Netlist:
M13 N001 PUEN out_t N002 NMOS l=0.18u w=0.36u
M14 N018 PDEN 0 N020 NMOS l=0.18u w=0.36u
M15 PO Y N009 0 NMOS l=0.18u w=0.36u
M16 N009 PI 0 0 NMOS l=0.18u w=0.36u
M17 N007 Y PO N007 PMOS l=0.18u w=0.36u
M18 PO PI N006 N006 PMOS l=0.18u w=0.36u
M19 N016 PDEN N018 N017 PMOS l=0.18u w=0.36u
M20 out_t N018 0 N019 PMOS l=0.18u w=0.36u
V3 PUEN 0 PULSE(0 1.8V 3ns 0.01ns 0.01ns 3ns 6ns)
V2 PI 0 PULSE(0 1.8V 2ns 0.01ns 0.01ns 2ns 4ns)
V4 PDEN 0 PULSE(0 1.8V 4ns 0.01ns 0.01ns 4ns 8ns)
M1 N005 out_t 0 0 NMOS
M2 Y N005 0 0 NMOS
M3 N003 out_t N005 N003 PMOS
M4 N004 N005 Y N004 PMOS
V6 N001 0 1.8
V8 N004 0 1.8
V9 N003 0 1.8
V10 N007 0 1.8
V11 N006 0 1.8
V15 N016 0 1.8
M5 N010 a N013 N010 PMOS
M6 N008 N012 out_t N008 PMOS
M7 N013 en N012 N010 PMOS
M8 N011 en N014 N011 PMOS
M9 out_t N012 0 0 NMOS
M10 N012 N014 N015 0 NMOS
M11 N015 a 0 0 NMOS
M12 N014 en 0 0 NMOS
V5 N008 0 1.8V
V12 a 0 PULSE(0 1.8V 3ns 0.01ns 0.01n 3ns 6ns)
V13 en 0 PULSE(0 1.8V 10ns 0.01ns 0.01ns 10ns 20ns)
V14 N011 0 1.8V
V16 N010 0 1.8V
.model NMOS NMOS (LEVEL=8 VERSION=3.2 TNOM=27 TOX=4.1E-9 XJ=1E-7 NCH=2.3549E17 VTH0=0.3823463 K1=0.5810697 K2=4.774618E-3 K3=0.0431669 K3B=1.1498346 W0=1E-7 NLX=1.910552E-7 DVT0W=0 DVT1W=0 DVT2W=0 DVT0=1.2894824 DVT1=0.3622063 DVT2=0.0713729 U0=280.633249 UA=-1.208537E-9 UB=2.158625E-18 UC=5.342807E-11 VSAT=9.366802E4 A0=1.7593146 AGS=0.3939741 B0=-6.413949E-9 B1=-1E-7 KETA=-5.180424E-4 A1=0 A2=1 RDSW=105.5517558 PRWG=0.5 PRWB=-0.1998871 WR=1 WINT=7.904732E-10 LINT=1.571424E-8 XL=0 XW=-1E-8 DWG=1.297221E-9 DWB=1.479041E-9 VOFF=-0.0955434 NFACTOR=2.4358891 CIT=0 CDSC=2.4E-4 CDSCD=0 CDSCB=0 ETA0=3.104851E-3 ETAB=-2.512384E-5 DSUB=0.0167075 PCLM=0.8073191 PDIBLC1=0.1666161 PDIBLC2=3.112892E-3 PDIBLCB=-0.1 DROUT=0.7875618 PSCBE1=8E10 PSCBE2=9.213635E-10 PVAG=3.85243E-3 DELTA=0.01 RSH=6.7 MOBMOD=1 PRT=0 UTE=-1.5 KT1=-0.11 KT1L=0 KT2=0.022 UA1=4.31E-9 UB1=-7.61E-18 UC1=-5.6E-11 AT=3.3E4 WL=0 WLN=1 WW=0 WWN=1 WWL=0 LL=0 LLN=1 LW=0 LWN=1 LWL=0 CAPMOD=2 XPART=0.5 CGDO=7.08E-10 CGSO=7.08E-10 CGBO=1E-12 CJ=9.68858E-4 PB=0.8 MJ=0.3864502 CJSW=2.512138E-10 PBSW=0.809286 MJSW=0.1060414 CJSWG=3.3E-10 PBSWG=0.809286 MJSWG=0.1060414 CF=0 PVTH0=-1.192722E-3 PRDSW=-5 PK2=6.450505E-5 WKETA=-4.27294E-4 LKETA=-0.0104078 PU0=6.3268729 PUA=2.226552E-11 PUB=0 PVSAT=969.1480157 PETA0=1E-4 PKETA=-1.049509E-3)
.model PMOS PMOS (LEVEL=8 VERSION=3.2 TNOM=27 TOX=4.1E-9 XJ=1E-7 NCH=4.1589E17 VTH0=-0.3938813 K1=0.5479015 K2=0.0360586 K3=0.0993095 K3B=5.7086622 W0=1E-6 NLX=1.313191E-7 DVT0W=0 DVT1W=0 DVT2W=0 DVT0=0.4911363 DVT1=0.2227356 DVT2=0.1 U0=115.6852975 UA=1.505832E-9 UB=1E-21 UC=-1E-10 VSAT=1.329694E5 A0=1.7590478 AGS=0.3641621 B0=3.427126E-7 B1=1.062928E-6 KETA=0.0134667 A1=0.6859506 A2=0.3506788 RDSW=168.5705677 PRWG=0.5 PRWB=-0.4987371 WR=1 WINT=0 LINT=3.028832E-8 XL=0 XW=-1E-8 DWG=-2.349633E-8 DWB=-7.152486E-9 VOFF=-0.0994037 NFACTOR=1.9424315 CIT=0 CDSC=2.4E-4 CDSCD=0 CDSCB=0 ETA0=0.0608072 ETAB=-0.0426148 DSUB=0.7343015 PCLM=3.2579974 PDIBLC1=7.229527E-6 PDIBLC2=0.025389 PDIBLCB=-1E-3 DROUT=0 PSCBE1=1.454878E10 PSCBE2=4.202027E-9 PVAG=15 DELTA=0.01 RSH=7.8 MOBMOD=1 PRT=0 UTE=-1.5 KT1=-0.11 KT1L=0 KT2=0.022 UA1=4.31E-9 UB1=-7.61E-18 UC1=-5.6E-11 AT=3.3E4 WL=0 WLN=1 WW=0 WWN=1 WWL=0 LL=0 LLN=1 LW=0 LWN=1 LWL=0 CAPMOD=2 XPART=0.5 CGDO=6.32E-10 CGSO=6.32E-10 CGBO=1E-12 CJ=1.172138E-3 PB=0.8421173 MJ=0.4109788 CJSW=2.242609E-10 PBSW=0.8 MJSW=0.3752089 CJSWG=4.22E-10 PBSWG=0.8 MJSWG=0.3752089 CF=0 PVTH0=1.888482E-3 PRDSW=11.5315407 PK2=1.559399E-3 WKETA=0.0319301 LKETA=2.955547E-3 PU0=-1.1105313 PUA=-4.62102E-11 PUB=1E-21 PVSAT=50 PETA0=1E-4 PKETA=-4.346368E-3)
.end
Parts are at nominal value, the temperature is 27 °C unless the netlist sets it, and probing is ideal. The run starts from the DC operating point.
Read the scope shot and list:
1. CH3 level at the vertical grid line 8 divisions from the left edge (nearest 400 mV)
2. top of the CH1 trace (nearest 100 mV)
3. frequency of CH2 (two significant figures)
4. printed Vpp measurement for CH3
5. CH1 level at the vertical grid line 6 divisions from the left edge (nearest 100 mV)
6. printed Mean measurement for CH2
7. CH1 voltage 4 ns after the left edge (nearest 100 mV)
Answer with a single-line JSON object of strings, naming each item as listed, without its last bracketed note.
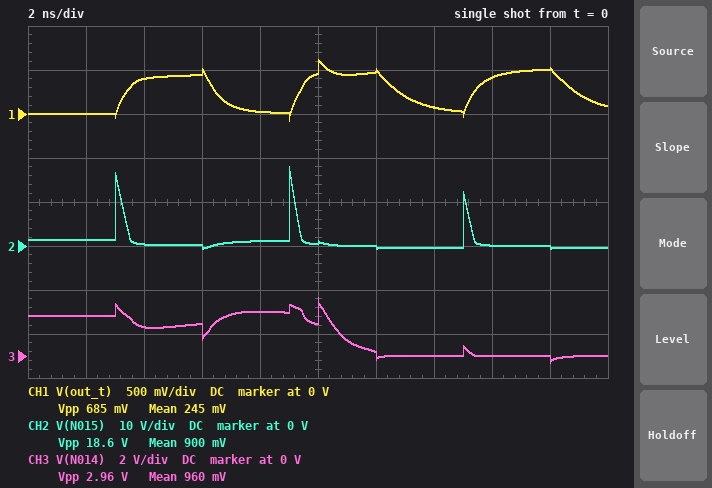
{"CH3 level at the vertical grid line 8 divisions from the left edge": "0 V", "top of the CH1 trace": "600 mV", "frequency of CH2": "170 MHz", "printed Vpp measurement for CH3": "2.96 V", "CH1 level at the vertical grid line 6 divisions from the left edge": "500 mV", "printed Mean measurement for CH2": "900 mV", "CH1 voltage 4 ns after the left edge": "400 mV"}
